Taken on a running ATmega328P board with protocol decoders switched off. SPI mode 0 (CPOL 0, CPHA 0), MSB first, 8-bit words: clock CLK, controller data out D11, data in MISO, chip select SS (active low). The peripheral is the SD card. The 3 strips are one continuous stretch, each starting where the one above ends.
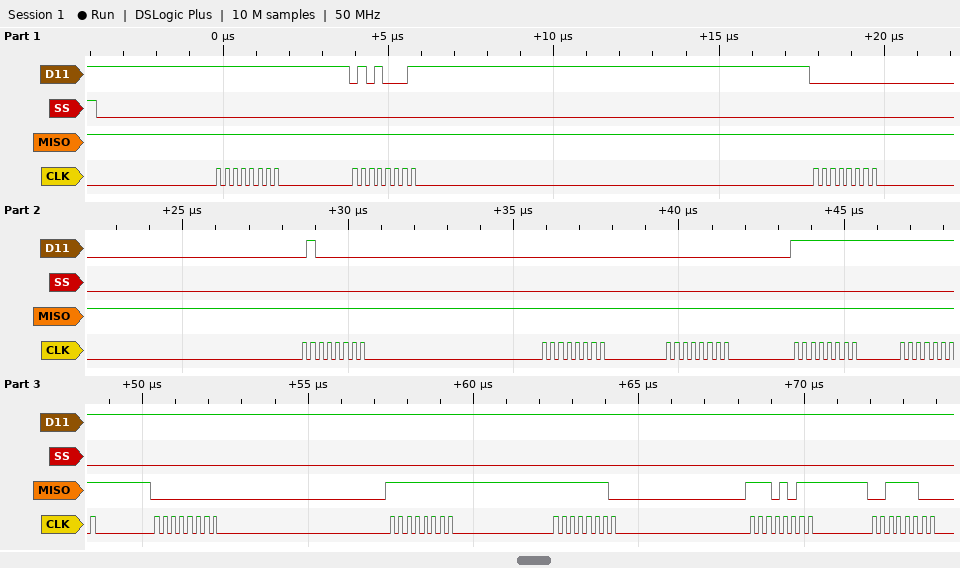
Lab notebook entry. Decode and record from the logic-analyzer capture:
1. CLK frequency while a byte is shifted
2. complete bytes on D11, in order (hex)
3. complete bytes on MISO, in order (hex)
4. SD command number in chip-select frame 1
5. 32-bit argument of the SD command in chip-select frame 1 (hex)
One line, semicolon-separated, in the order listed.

4 MHz; 0xFF 0x51 0x00 0x40 0x00 0x00 0xFF 0xFF 0xFF 0xFF 0xFF 0xFF 0xFF; 0xFF 0xFF 0xFF 0xFF 0xFF 0xFF 0xFF 0xFF 0x00 0xFF 0xFE 0xEB 0x3C; CMD17; 0x00400000
